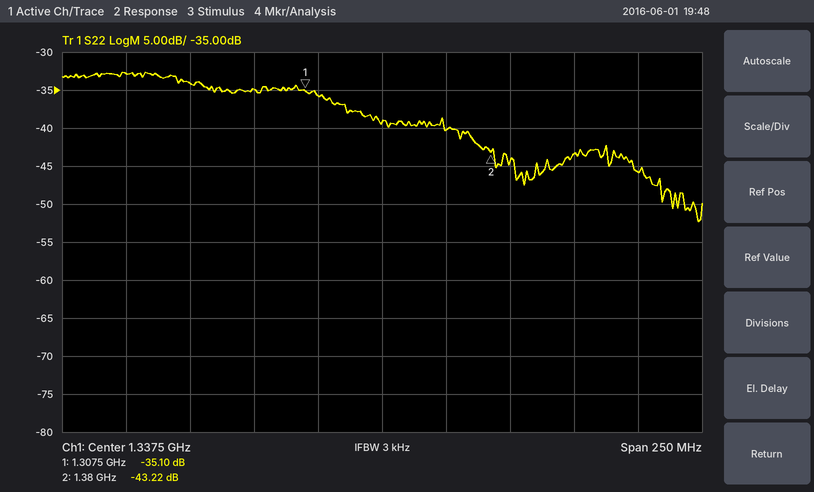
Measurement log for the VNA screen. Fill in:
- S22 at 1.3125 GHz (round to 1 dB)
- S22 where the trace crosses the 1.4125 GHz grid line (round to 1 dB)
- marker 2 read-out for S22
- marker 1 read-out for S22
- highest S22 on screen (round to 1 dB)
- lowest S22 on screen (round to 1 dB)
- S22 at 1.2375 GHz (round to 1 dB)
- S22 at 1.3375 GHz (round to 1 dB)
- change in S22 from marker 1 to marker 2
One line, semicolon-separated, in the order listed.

-36 dB; -43 dB; -43.22 dB; -35.10 dB; -33 dB; -52 dB; -33 dB; -39 dB; -8.12 dB
